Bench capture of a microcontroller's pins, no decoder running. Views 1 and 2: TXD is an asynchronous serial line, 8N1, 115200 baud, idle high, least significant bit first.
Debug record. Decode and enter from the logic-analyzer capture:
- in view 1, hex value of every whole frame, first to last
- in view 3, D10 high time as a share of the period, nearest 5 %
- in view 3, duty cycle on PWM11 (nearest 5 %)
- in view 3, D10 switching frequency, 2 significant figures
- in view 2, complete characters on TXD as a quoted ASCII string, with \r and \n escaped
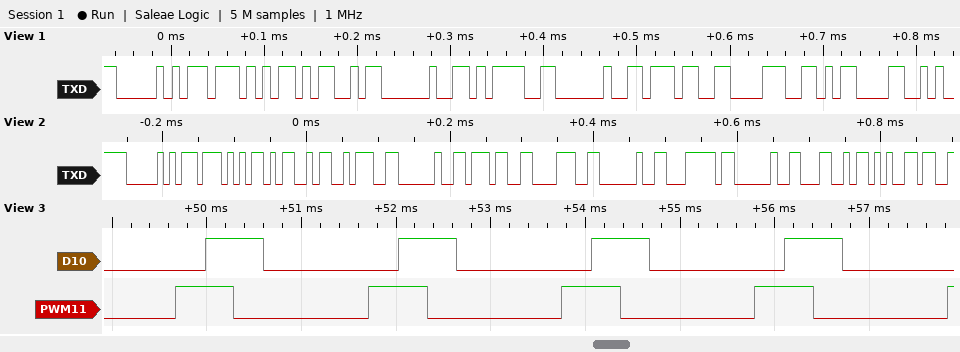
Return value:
0x50 0x57 0x4D 0x20 0x3D 0x20 0x37 0x38 0x0D
30 %
30 %
490 Hz
"PWM: 78 | Le"
